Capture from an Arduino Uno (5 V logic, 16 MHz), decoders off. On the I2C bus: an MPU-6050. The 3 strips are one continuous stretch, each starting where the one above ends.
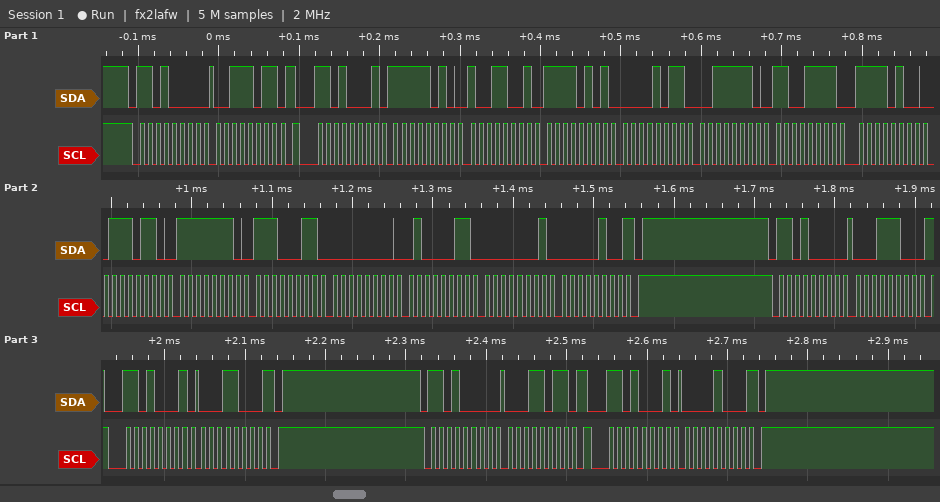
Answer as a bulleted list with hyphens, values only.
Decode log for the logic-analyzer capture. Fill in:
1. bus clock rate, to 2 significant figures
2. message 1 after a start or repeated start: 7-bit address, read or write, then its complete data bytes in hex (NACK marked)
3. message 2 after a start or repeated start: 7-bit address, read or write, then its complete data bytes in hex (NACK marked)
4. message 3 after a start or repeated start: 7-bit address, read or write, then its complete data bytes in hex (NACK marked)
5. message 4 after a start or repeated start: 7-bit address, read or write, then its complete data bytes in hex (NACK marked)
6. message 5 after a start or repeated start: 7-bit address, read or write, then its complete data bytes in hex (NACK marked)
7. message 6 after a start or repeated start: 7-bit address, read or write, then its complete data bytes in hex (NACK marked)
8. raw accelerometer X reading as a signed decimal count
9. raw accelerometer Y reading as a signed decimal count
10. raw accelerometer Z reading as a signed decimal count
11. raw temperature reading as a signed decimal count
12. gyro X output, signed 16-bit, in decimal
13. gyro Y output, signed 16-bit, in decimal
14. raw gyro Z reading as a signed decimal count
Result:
- 100 kHz
- 0x68 write: 3B
- 0x68 read: FA 99 F5 0B 3E CF F4 76 FE E3 00 43 01 04 NACK
- 0x68 write: 1C
- 0x68 read: 18 NACK
- 0x68 write: 1B
- 0x68 read: 08 NACK
- -1383
- -2805
- 16079
- -2954
- -285
- 67
- 260
